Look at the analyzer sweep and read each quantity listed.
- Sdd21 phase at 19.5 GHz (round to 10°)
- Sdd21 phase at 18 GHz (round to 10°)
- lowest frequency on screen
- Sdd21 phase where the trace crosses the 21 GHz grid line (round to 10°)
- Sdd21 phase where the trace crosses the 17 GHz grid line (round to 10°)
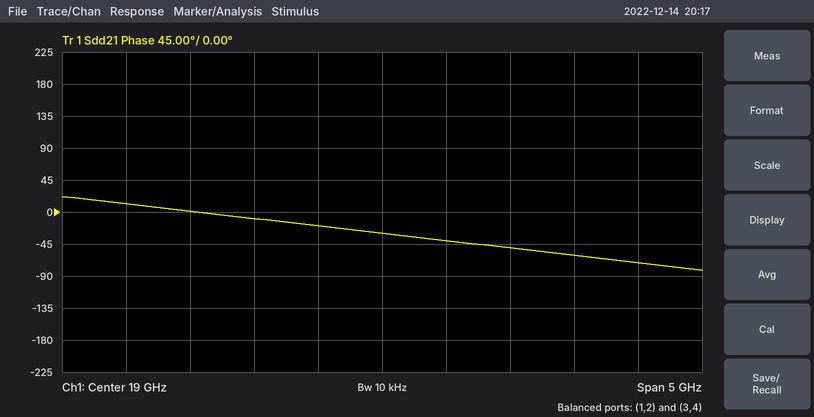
-40°
-10°
16.5 GHz
-70°
10°
